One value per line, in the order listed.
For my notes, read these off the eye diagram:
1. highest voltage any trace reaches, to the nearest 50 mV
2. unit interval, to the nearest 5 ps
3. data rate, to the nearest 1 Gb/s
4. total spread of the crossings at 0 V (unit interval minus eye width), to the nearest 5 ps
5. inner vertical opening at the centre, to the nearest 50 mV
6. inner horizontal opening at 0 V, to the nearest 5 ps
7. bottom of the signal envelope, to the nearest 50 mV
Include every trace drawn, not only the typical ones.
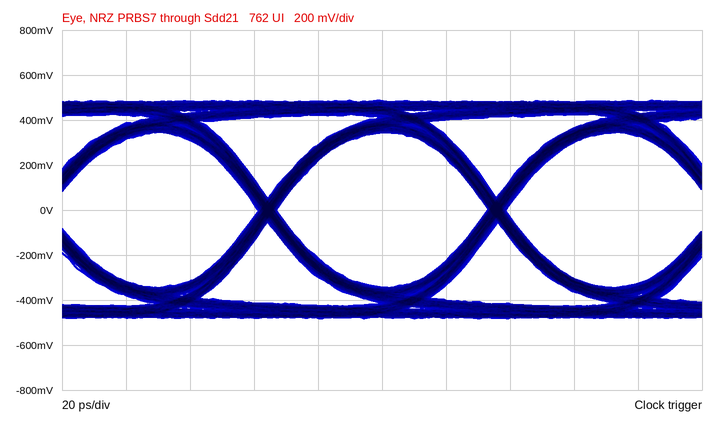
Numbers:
500 mV
70 ps
14 Gb/s
5 ps
700 mV
65 ps
-500 mV
